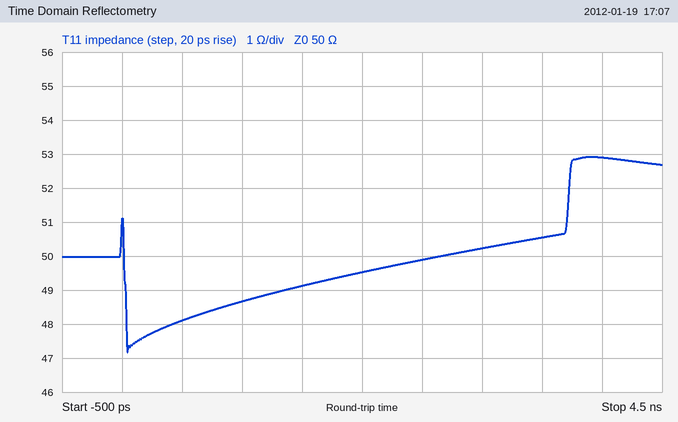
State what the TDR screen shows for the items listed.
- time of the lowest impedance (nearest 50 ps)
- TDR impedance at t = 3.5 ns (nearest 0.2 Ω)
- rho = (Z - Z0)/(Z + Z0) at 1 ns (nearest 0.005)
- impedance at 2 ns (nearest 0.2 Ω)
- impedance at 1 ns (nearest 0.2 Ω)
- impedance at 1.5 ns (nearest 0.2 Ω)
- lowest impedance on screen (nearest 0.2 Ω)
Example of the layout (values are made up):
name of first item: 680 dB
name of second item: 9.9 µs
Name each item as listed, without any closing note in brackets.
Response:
time of the lowest impedance: 50 ps
TDR impedance at t = 3.5 ns: 50.6 Ω
rho = (Z - Z0)/(Z + Z0) at 1 ns: -0.015
impedance at 2 ns: 49.6 Ω
impedance at 1 ns: 48.6 Ω
impedance at 1.5 ns: 49.2 Ω
lowest impedance on screen: 47.2 Ω
